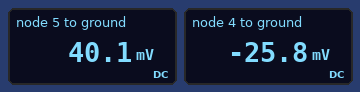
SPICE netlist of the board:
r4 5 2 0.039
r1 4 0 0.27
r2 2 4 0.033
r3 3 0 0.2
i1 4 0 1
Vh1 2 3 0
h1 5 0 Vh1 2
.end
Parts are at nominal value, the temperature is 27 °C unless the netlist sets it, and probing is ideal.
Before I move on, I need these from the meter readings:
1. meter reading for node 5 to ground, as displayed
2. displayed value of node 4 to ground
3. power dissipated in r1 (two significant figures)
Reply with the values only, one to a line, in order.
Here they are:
40.1 mV
-25.8 mV
2.5 mW
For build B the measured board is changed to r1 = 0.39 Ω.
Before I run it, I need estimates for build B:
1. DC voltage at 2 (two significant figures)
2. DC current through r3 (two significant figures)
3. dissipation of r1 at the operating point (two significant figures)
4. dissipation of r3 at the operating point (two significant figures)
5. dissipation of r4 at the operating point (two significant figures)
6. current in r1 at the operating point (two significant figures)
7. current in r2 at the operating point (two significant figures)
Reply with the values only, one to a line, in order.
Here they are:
4.1 mV
21 mA
1.8 mW
85 µW
35 mW
68 mA
930 mA
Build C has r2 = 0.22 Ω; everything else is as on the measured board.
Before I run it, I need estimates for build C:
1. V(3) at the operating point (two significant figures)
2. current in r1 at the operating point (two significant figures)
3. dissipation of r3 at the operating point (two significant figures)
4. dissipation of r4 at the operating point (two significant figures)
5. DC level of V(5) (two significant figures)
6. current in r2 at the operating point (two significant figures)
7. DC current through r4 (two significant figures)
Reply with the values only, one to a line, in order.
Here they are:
2.5 mV
440 mA
30 µW
13 mW
25 mV
560 mA
570 mA
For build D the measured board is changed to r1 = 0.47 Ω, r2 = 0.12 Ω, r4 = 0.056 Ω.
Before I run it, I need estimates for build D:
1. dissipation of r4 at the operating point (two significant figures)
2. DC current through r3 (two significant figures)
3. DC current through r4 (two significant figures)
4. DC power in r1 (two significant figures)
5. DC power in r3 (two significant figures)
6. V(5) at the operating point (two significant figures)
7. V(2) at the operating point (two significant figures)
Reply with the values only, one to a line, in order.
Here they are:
39 mW
26 mA
830 mA
18 mW
130 µW
52 mV
5.2 mV
